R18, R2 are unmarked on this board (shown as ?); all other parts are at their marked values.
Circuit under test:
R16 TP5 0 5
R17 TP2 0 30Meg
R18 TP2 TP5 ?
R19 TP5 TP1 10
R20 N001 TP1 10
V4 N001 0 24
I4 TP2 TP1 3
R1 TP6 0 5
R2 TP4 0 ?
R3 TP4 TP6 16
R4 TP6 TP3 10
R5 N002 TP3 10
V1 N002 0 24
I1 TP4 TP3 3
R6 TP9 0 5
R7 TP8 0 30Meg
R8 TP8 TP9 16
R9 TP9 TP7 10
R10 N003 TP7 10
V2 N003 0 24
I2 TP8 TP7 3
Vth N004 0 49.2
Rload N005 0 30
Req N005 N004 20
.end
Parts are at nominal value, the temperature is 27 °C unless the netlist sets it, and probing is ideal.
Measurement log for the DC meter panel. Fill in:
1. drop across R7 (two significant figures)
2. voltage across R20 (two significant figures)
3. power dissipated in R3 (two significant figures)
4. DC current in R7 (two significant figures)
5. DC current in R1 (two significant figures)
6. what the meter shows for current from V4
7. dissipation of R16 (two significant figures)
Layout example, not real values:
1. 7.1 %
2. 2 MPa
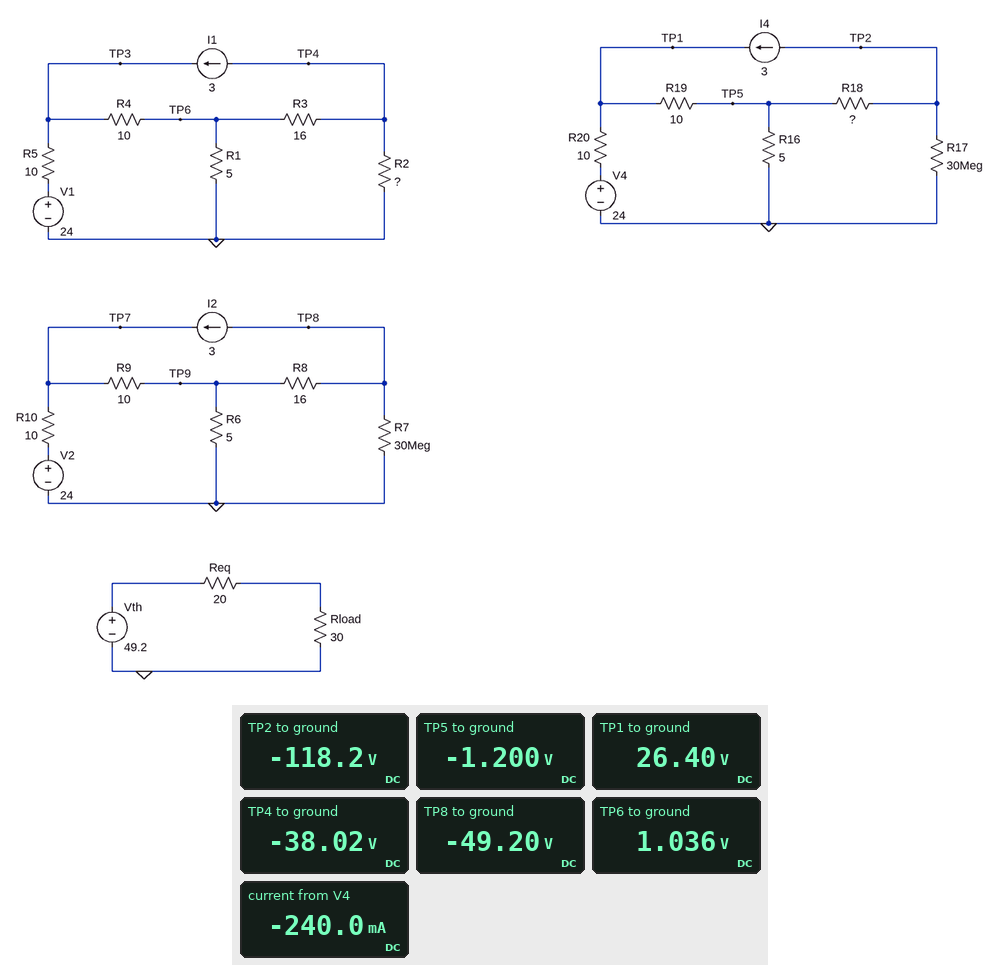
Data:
1. 49 V
2. 2.4 V
3. 95 W
4. 1.6 µA
5. 210 mA
6. -240.0 mA
7. 290 mW
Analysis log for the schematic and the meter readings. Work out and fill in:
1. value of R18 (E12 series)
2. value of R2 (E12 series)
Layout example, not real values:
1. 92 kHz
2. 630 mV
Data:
1. 39 Ω
2. 68 Ω
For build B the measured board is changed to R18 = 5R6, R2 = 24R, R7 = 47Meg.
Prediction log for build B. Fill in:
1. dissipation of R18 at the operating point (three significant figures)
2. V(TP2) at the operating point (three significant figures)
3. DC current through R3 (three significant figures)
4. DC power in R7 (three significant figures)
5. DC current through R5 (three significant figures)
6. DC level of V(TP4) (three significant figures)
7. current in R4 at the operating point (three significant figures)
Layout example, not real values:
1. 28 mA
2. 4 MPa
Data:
1. 50.4 W
2. -18.0 V
3. 1.88 A
4. 51.5 µW
5. 464 mA
6. -26.8 V
7. 2.54 A
